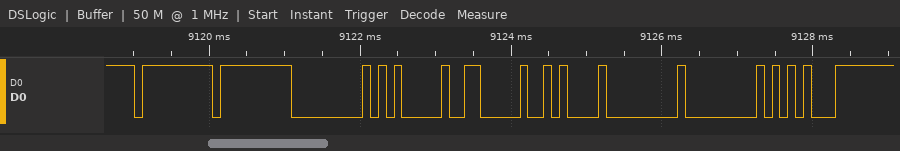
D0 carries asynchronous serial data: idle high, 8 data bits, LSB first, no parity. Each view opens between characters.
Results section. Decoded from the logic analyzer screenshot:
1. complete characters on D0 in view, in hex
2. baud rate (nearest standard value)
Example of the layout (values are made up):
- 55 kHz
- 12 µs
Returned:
- FF, FF, 00, 05, 06, 0A, 00, 00, 15
- 9600 baud
